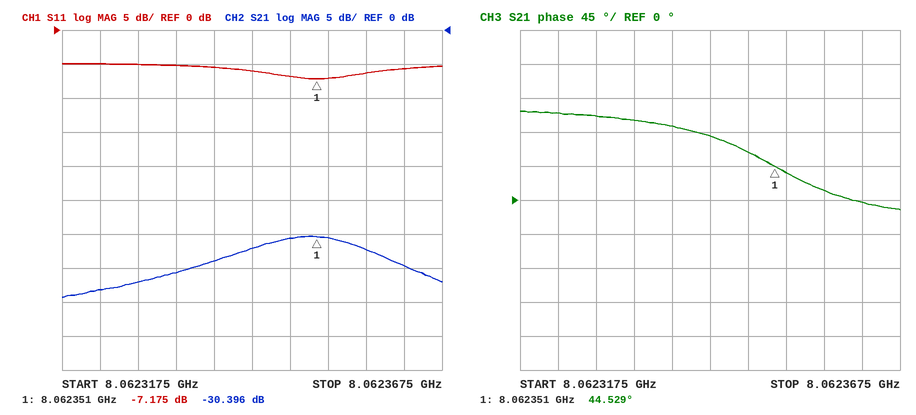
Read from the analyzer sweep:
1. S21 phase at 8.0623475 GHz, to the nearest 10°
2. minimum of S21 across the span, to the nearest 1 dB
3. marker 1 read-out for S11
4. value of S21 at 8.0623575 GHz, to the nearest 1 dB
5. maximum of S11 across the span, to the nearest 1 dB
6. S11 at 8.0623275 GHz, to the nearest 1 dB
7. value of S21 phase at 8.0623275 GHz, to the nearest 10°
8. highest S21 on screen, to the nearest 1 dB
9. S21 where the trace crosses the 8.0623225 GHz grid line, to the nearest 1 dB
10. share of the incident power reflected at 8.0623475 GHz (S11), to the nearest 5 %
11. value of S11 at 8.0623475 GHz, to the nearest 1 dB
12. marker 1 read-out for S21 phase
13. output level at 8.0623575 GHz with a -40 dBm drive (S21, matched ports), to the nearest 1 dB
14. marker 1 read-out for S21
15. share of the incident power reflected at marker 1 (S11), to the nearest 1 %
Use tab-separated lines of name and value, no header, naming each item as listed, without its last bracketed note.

S21 phase at 8.0623475 GHz, to the nearest 10°	60°
minimum of S21 across the span, to the nearest 1 dB	-39 dB
marker 1 read-out for S11	-7.175 dB
value of S21 at 8.0623575 GHz, to the nearest 1 dB	-32 dB
maximum of S11 across the span, to the nearest 1 dB	-5 dB
S11 at 8.0623275 GHz, to the nearest 1 dB	-5 dB
value of S21 phase at 8.0623275 GHz, to the nearest 10°	110°
highest S21 on screen, to the nearest 1 dB	-30 dB
S21 where the trace crosses the 8.0623225 GHz grid line, to the nearest 1 dB	-38 dB
share of the incident power reflected at 8.0623475 GHz (S11), to the nearest 5 %	20 %
value of S11 at 8.0623475 GHz, to the nearest 1 dB	-7 dB
marker 1 read-out for S21 phase	44.529°
output level at 8.0623575 GHz with a -40 dBm drive (S21, matched ports), to the nearest 1 dB	-72 dBm
marker 1 read-out for S21	-30.396 dB
share of the incident power reflected at marker 1 (S11), to the nearest 1 %	19 %
